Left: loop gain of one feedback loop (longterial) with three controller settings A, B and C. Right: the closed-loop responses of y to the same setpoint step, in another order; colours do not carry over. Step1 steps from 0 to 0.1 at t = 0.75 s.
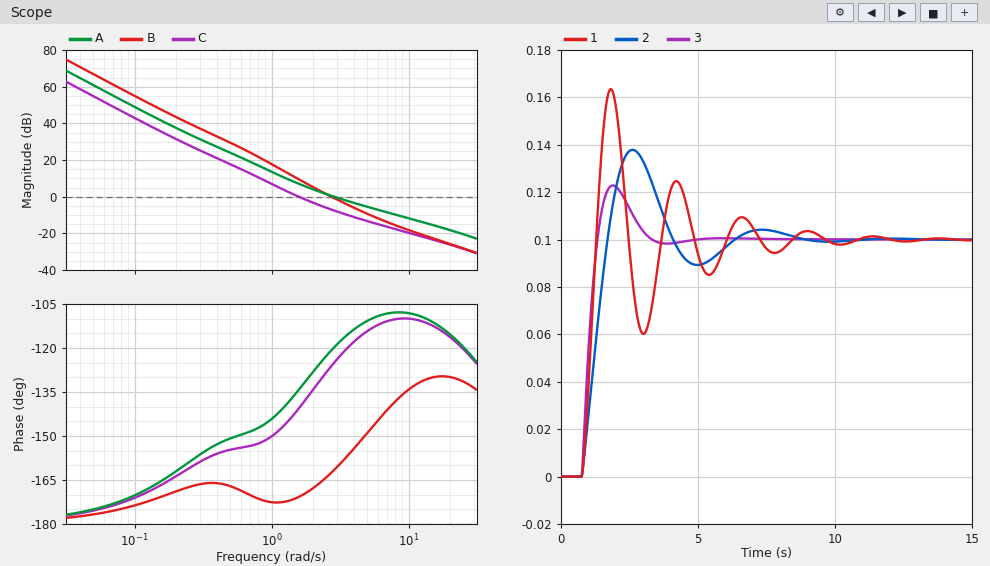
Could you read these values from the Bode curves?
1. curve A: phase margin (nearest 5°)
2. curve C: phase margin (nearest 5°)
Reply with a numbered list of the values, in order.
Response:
1. 60°
2. 40°
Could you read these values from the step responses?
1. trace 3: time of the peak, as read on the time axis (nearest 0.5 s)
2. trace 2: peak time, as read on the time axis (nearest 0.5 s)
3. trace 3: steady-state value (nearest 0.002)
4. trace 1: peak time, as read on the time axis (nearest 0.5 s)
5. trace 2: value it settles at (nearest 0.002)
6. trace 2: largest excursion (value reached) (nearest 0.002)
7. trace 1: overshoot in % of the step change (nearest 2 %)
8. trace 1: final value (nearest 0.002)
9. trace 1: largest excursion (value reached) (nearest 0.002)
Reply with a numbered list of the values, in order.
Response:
1. 2.0 s
2. 2.5 s
3. 0.100
4. 2.0 s
5. 0.100
6. 0.138
7. 64 %
8. 0.100
9. 0.164
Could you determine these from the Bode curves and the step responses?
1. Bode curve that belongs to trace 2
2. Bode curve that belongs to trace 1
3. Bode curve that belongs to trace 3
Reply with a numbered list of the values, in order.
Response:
1. C
2. B
3. A
